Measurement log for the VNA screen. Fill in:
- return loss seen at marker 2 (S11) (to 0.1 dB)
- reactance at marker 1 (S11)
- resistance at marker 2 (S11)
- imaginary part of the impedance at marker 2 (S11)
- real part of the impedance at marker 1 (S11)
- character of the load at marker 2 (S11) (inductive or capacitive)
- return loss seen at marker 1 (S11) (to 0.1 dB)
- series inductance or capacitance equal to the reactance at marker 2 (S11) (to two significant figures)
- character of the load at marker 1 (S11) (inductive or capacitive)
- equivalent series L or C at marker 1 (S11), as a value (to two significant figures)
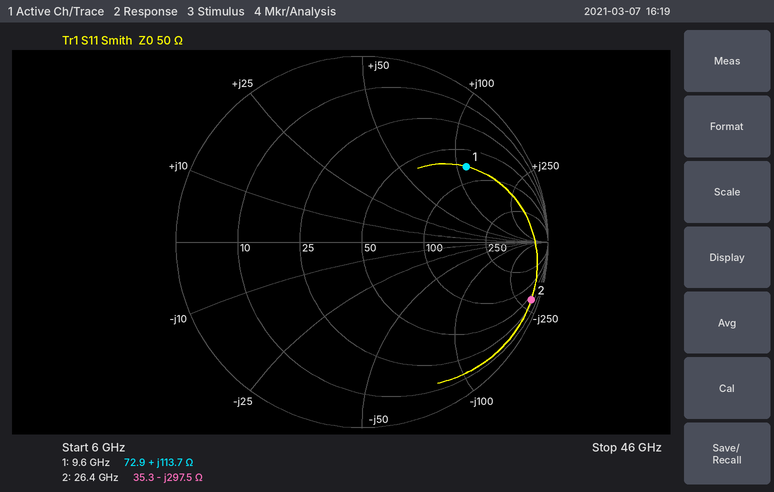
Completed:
0.3 dB
+113.7 Ω
35.3 Ω
-297.5 Ω
72.9 Ω
capacitive
3.2 dB
20 fF
inductive
1.9 nH
